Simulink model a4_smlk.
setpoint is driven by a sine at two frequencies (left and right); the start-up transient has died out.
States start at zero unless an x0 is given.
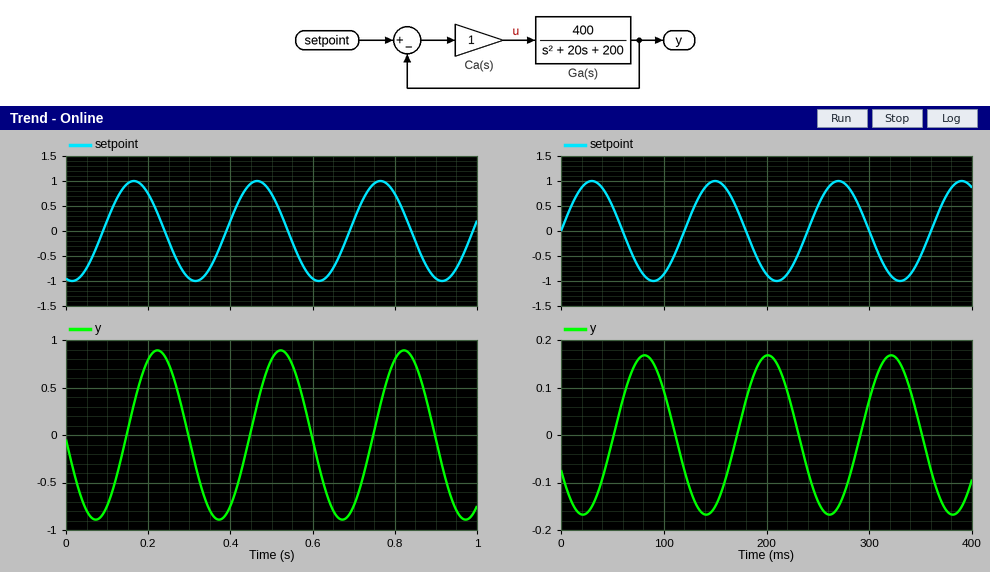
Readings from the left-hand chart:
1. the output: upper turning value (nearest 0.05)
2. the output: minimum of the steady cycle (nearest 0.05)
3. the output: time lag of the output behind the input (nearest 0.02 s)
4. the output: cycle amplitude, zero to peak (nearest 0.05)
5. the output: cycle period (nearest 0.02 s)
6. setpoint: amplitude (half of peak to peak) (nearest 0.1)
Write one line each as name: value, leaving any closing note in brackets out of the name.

the output: upper turning value: 0.90
the output: minimum of the steady cycle: -0.90
the output: time lag of the output behind the input: 0.06 s
the output: cycle amplitude, zero to peak: 0.90
the output: cycle period: 0.30 s
setpoint: amplitude (half of peak to peak): 1.0
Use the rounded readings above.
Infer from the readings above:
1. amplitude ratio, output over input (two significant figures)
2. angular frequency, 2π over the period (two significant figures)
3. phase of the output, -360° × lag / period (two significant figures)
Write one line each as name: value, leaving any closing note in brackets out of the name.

amplitude ratio, output over input: 0.90
angular frequency, 2π over the period: 21 rad/s
phase of the output, -360° × lag / period: -72°
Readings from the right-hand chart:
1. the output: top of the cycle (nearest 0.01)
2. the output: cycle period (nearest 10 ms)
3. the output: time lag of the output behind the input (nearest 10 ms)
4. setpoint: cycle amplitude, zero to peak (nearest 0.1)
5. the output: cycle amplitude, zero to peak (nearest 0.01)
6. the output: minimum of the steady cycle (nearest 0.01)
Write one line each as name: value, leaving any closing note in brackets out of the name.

the output: top of the cycle: 0.17
the output: cycle period: 120 ms
the output: time lag of the output behind the input: 50 ms
setpoint: cycle amplitude, zero to peak: 1.0
the output: cycle amplitude, zero to peak: 0.17
the output: minimum of the steady cycle: -0.17
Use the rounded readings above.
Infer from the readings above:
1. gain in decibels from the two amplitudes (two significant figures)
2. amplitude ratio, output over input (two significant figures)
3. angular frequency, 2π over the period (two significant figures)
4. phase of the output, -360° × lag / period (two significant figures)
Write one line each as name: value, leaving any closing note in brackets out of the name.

gain in decibels from the two amplitudes: -15 dB
amplitude ratio, output over input: 0.17
angular frequency, 2π over the period: 0.052 rad/ms
phase of the output, -360° × lag / period: -150°
